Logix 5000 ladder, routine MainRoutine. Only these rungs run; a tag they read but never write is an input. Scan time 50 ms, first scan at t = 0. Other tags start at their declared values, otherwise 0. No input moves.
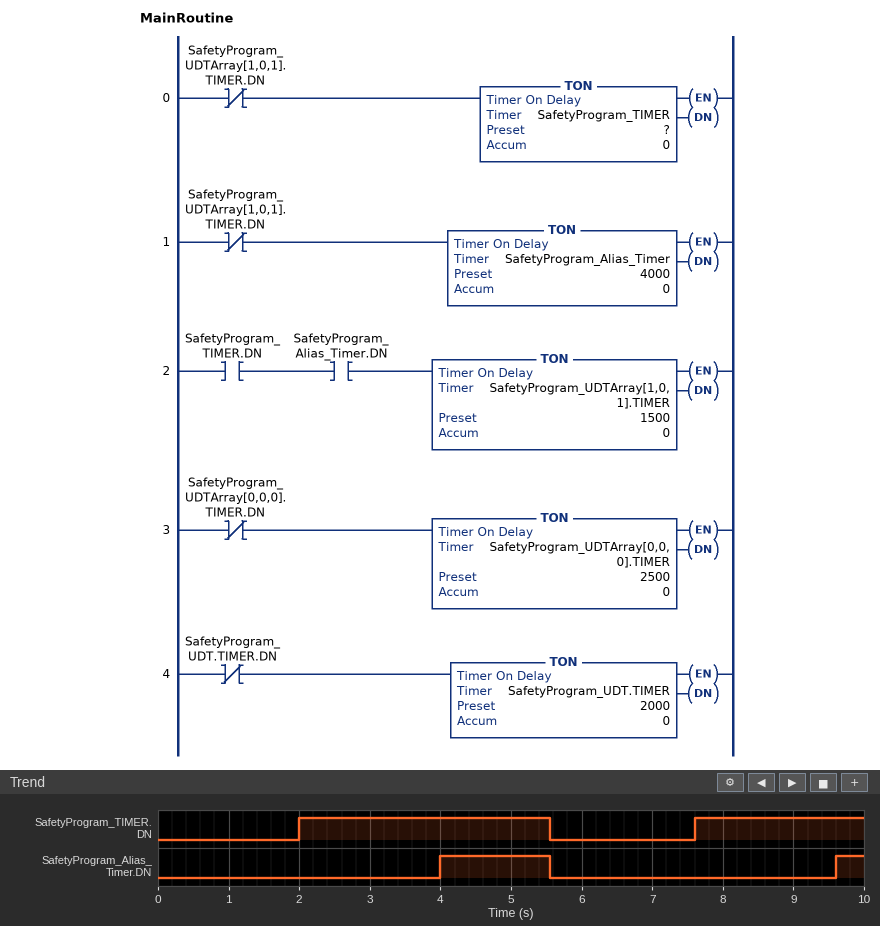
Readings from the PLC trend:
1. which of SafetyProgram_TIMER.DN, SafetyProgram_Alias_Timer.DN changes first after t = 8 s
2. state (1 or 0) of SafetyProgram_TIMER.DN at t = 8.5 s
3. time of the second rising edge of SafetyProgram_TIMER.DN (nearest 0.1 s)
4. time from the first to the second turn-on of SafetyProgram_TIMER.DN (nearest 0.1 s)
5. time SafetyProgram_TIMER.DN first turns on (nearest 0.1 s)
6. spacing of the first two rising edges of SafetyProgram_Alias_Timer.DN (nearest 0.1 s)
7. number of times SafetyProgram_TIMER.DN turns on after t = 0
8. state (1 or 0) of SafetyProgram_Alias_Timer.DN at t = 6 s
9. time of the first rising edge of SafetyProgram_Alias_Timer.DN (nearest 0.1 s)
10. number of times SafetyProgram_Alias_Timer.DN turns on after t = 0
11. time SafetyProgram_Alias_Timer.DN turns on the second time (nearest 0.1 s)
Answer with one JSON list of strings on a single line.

["SafetyProgram_Alias_Timer.DN", "1", "7.6 s", "5.6 s", "2.0 s", "5.6 s", "2", "0", "4.0 s", "2", "9.6 s"]
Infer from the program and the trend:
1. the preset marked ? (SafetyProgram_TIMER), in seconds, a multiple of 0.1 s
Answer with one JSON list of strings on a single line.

["2.0 s"]
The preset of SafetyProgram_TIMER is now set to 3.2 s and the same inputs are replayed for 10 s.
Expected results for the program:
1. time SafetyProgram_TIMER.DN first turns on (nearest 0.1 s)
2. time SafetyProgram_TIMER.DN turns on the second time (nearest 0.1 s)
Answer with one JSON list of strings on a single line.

["3.2 s", "8.8 s"]
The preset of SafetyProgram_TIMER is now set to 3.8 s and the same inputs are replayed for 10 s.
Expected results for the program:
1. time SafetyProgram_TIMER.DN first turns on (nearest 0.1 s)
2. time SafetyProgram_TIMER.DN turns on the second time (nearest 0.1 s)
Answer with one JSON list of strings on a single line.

["3.8 s", "9.4 s"]
